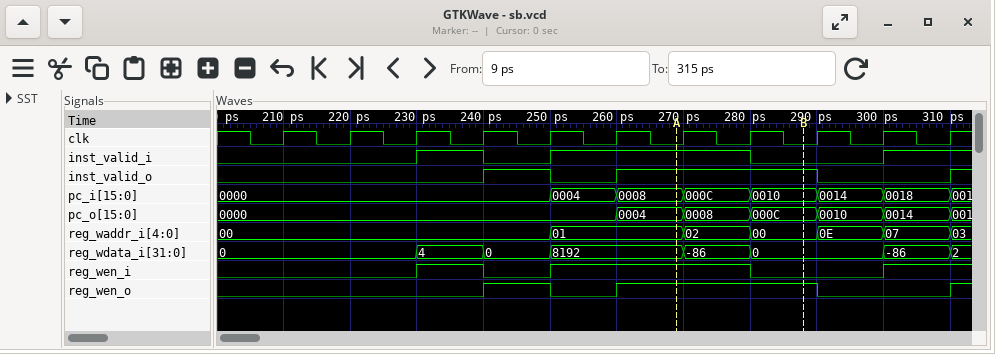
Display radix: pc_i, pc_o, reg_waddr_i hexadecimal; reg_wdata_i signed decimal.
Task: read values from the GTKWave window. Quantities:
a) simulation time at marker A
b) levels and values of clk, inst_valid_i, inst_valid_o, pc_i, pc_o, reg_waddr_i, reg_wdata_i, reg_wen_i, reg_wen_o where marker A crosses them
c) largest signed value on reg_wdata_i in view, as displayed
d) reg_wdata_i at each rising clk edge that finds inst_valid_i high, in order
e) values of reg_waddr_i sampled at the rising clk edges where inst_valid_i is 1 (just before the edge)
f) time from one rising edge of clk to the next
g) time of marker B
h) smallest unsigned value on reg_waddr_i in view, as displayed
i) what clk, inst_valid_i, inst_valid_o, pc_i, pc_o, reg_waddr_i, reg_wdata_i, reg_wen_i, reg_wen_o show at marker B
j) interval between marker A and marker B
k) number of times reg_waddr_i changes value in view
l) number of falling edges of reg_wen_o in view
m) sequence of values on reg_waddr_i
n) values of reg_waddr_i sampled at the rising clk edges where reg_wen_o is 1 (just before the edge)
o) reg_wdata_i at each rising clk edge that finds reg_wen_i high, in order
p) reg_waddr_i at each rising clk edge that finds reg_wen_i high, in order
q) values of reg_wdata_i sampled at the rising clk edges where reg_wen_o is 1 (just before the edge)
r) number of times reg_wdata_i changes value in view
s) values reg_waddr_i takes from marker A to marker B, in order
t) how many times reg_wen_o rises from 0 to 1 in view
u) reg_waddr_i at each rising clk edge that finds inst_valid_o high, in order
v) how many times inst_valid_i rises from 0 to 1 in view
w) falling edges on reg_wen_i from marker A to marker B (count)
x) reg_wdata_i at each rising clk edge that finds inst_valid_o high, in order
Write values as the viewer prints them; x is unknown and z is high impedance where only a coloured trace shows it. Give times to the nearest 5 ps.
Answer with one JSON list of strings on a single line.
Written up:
["270 ps", "clk=0, inst_valid_i=1, inst_valid_o=1, pc_i=0008, pc_o=0004, reg_waddr_i=01, reg_wdata_i=8192, reg_wen_i=1, reg_wen_o=1", "8192", "4, 8192, 8192, -86, -86", "00, 01, 01, 02, 07", "10 ps", "290 ps", "00", "clk=0, inst_valid_i=0, inst_valid_o=1, pc_i=0010, pc_o=000C, reg_waddr_i=00, reg_wdata_i=0, reg_wen_i=0, reg_wen_o=1", "20 ps", "6", "2", "00, 01, 02, 00, 0E, 07, 03", "00, 01, 02, 00", "4, 8192, 8192, -86, -86", "00, 01, 01, 02, 07", "0, 8192, -86, 0", "7", "01, 02, 00", "3", "00, 01, 02, 00", "3", "1", "0, 8192, -86, 0"]
